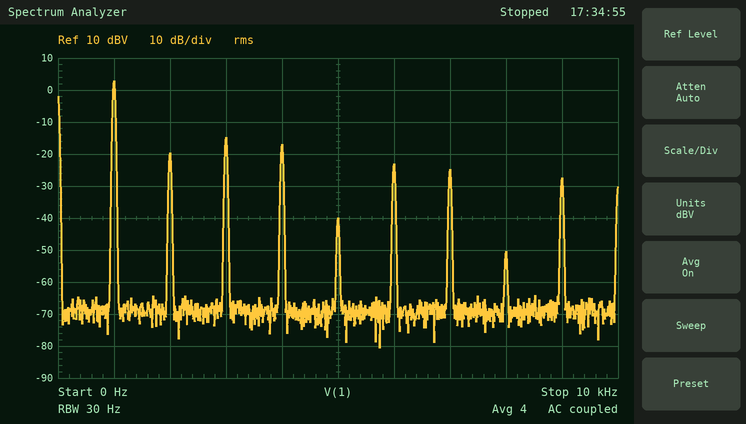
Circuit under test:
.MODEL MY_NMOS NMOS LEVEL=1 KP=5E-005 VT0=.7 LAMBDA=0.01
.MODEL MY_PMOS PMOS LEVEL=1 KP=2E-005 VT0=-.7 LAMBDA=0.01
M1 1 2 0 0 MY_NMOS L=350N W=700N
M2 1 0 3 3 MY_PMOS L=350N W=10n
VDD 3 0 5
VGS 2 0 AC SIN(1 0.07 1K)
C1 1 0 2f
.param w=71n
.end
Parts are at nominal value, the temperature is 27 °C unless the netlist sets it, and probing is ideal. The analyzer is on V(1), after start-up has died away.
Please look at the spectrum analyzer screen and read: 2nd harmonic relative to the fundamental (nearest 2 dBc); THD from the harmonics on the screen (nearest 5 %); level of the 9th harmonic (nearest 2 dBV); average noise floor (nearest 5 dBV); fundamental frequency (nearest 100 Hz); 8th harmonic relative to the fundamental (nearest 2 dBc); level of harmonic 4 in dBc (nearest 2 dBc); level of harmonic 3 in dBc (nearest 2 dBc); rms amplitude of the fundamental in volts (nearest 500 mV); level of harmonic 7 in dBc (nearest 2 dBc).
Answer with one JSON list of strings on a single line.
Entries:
["-22 dBc", "20 %", "-28 dBV", "-70 dBV", "1.0 kHz", "-54 dBc", "-20 dBc", "-18 dBc", "1.5 V", "-28 dBc"]
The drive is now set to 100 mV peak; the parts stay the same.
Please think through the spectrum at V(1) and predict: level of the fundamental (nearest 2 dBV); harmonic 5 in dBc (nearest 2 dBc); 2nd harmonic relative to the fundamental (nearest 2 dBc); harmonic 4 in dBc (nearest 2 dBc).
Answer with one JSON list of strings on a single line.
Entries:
["4 dBV", "-26 dBc", "-46 dBc", "-24 dBc"]
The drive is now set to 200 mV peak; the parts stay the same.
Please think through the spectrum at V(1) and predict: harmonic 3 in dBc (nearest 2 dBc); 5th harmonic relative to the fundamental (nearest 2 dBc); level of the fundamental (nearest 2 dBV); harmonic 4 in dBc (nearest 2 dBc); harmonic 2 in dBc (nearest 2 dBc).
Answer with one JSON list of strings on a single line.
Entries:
["-14 dBc", "-20 dBc", "6 dBV", "-50 dBc", "-22 dBc"]
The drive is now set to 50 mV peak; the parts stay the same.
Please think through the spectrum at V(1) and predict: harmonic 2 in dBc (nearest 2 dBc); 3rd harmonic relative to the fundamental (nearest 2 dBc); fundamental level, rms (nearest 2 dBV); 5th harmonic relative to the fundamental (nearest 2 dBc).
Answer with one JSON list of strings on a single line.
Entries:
["-16 dBc", "-28 dBc", "2 dBV", "-24 dBc"]
